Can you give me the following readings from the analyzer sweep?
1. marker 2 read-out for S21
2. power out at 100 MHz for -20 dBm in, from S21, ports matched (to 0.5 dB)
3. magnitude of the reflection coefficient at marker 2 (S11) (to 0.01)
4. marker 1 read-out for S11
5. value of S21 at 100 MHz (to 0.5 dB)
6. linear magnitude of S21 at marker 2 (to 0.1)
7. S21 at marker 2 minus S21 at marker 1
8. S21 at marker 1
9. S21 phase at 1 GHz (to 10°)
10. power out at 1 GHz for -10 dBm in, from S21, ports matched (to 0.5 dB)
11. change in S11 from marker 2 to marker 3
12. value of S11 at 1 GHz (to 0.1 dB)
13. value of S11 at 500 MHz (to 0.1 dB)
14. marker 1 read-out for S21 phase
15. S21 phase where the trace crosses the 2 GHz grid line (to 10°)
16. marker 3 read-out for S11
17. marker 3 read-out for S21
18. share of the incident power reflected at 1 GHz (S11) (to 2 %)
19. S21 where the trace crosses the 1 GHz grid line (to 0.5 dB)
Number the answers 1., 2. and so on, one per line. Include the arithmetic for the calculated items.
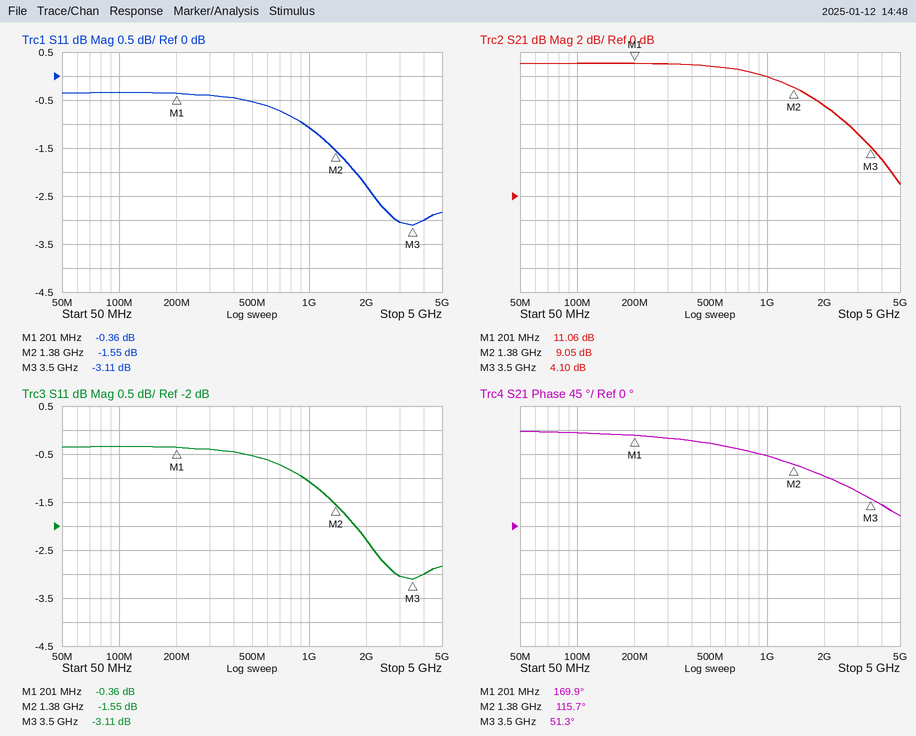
1. 9.05 dB
2. -20 dBm + (11.0 dB) = -9.0 dBm
3. 10^(-1.55/20) ≈ 0.84
4. -0.36 dB
5. 11.0 dB
6. 10^(9.05/20) ≈ 2.8
7. 9.05 − (11.06) = -2.01 dB
8. 11.06 dB
9. 130°
10. -10 dBm + (10.0 dB) = 0.0 dBm
11. -3.11 − (-1.55) = -1.56 dB
12. -1.1 dB
13. -0.5 dB
14. 169.9°
15. 90°
16. -3.11 dB
17. 4.10 dB
18. 10^(-1.1/10) ≈ 78 %
19. 10.0 dB
